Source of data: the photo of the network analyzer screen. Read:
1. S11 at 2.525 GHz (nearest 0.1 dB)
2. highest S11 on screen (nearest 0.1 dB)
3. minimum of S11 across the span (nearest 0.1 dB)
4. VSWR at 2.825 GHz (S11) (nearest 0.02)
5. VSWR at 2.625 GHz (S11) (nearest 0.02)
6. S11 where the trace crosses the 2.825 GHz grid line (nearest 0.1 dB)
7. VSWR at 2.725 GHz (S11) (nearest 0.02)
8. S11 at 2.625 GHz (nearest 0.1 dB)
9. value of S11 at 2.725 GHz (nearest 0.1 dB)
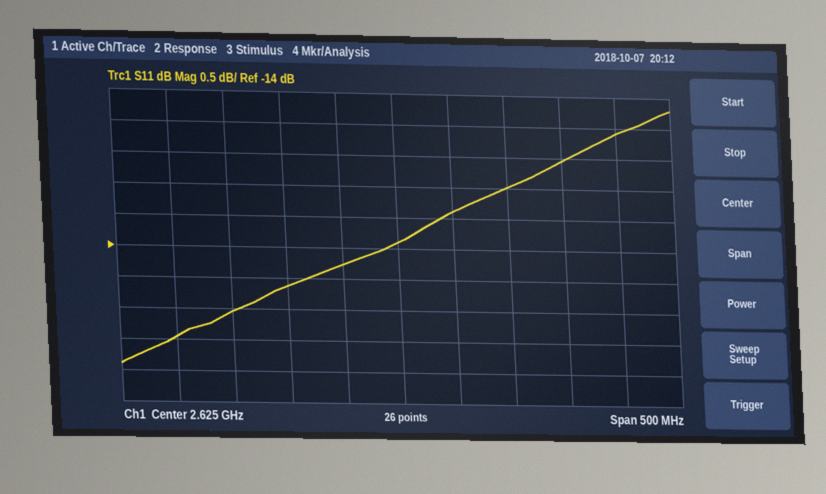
-14.6 dB
-11.7 dB
-15.9 dB
1.66
1.50
-12.1 dB
1.58
-13.9 dB
-13.0 dB
